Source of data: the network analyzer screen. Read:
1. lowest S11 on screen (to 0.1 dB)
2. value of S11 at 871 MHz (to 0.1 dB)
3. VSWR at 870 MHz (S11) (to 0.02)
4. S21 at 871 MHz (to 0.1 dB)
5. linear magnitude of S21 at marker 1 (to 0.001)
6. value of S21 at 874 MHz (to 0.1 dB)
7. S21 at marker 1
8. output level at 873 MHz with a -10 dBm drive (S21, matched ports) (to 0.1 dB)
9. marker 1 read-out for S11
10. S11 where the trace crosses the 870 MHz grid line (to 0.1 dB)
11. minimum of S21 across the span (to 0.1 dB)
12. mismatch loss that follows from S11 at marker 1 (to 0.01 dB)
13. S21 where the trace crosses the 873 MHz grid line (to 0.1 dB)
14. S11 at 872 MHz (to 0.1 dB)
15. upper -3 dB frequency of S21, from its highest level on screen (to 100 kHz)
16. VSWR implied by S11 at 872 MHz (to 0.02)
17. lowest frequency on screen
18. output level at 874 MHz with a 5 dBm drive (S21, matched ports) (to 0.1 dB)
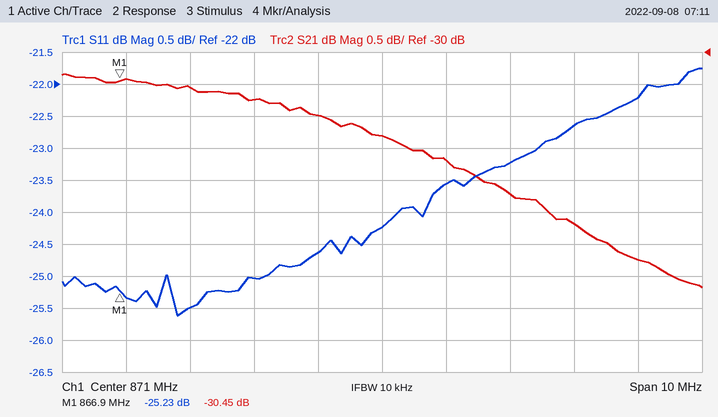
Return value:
-25.6 dB
-24.2 dB
1.12
-31.3 dB
0.030
-32.7 dB
-30.45 dB
-42.2 dBm
-25.23 dB
-24.6 dB
-33.7 dB
0.01 dB
-32.2 dB
-23.6 dB
875.3 MHz
1.14
866 MHz
-27.7 dBm
